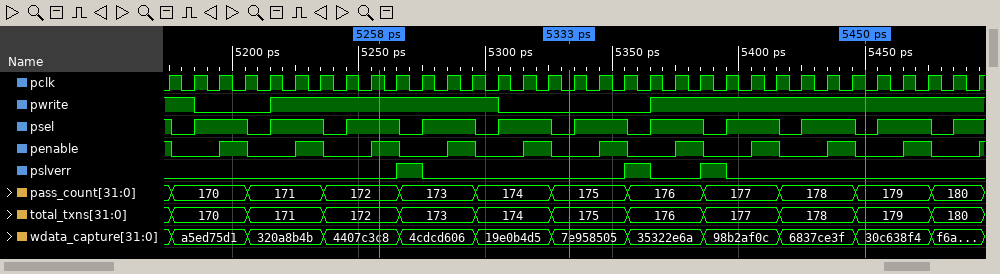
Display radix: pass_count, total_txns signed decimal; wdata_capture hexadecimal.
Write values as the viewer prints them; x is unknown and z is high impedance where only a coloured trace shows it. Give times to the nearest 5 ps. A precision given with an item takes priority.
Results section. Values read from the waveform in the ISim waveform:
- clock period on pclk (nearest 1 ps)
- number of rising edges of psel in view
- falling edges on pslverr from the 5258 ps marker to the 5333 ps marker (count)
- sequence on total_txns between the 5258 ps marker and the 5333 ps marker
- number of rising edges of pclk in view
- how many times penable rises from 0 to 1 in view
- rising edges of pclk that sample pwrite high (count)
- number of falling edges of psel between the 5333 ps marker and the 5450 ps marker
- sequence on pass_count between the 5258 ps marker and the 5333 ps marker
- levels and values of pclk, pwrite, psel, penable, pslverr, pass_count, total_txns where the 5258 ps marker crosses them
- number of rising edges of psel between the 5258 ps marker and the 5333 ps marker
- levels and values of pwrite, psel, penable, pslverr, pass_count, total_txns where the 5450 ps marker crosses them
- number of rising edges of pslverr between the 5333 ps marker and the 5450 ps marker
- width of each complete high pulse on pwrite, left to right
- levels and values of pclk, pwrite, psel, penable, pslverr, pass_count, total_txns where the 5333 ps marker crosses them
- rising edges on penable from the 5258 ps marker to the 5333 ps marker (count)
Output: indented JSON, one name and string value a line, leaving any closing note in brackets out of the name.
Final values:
{
  "clock period on pclk": "10 ps",
  "number of rising edges of psel in view": "11",
  "falling edges on pslverr from the 5258 ps marker to the 5333 ps marker": "1",
  "sequence on total_txns between the 5258 ps marker and the 5333 ps marker": "172, 173, 174, 175",
  "number of rising edges of pclk in view": "33",
  "how many times penable rises from 0 to 1 in view": "11",
  "rising edges of pclk that sample pwrite high": "24",
  "number of falling edges of psel between the 5333 ps marker and the 5450 ps marker": "4",
  "sequence on pass_count between the 5258 ps marker and the 5333 ps marker": "172, 173, 174, 175",
  "levels and values of pclk, pwrite, psel, penable, pslverr, pass_count, total_txns where the 5258 ps marker crosses them": "pclk=1, pwrite=1, psel=1, penable=1, pslverr=0, pass_count=172, total_txns=172",
  "number of rising edges of psel between the 5258 ps marker and the 5333 ps marker": "2",
  "levels and values of pwrite, psel, penable, pslverr, pass_count, total_txns where the 5450 ps marker crosses them": "pwrite=1, psel=0, penable=0, pslverr=0, pass_count=179, total_txns=179",
  "number of rising edges of pslverr between the 5333 ps marker and the 5450 ps marker": "2",
  "width of each complete high pulse on pwrite, left to right": "90 ps",
  "levels and values of pclk, pwrite, psel, penable, pslverr, pass_count, total_txns where the 5333 ps marker crosses them": "pclk=0, pwrite=0, psel=0, penable=0, pslverr=0, pass_count=175, total_txns=175",
  "rising edges on penable from the 5258 ps marker to the 5333 ps marker": "2"
}
